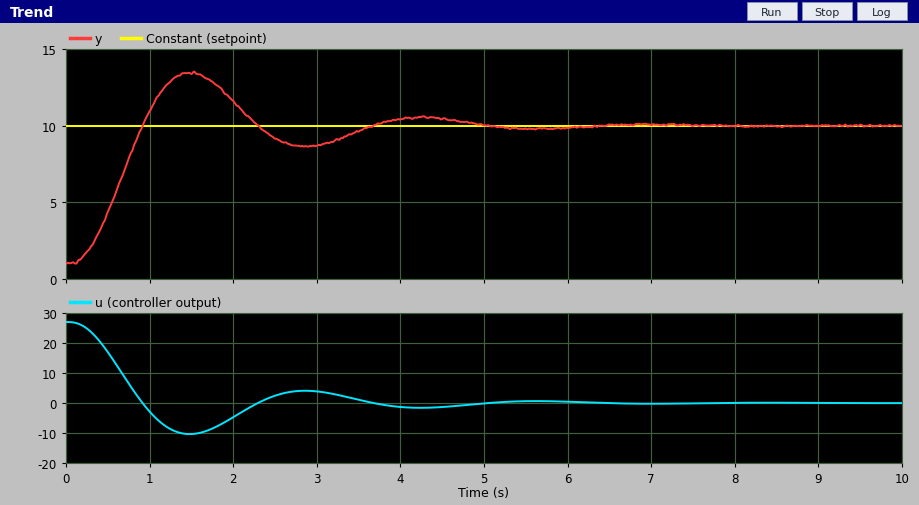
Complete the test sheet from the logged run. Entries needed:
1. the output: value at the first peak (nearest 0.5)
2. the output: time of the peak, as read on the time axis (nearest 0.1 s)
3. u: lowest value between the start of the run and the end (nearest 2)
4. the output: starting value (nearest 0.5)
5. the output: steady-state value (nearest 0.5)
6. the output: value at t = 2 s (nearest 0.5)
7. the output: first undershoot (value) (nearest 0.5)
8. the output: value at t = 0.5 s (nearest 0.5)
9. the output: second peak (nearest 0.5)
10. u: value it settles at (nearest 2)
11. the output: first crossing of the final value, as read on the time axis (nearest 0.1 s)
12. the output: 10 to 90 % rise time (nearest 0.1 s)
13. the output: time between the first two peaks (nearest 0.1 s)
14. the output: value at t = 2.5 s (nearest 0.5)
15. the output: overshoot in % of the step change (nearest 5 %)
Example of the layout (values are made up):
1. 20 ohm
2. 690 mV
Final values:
1. 13.5
2. 1.5 s
3. -10
4. 1.0
5. 10.0
6. 11.5
7. 8.5
8. 4.5
9. 10.5
10. 0
11. 0.9 s
12. 0.6 s
13. 2.8 s
14. 9.0
15. 40 %
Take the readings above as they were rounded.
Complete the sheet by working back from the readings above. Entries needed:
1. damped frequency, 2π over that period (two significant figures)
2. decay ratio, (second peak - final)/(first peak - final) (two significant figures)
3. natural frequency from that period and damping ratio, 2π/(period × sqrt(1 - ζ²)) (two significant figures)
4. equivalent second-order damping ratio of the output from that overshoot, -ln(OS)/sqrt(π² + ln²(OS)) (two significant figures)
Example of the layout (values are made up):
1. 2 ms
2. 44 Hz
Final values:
1. 2.2 rad/s
2. 0.14
3. 2.3 rad/s
4. 0.28
